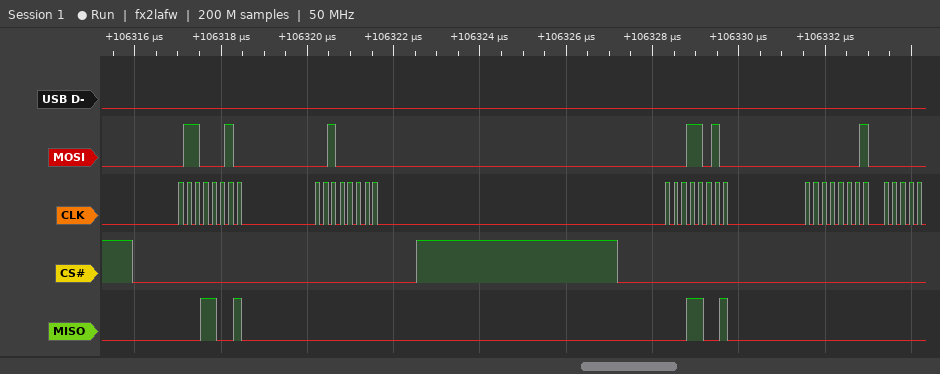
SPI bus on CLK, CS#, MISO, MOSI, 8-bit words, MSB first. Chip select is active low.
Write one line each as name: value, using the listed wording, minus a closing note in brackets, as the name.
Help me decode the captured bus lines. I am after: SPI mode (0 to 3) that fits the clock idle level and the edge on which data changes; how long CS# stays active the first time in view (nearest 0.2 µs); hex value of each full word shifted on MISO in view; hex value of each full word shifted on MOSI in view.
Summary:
SPI mode (0 to 3) that fits the clock idle level and the edge on which data changes: 0
how long CS# stays active the first time in view: 6.6 µs
hex value of each full word shifted on MISO in view: 19, 00, 19, 00
hex value of each full word shifted on MOSI in view: 62, 20, 1A, 01
